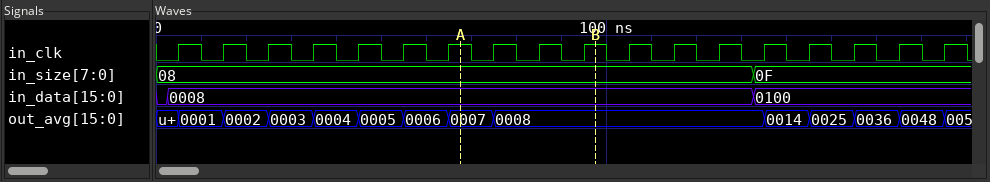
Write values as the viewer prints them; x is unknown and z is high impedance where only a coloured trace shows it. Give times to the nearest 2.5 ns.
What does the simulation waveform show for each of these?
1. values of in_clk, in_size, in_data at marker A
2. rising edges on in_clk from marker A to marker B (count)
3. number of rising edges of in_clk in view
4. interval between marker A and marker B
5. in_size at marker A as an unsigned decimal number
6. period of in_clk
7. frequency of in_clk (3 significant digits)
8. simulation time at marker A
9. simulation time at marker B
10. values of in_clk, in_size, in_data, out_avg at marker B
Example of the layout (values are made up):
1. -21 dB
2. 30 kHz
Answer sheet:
1. in_clk=1, in_size=08, in_data=0008
2. 3
3. 18
4. 30 ns
5. 8
6. 10 ns
7. 100 MHz
8. 67.5 ns
9. 97.5 ns
10. in_clk=1, in_size=08, in_data=0008, out_avg=0008
